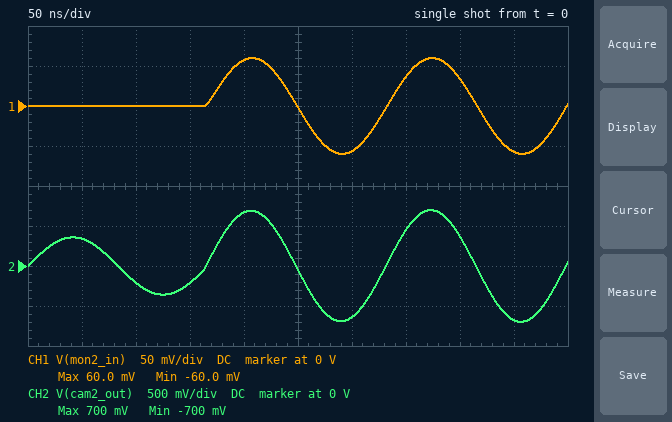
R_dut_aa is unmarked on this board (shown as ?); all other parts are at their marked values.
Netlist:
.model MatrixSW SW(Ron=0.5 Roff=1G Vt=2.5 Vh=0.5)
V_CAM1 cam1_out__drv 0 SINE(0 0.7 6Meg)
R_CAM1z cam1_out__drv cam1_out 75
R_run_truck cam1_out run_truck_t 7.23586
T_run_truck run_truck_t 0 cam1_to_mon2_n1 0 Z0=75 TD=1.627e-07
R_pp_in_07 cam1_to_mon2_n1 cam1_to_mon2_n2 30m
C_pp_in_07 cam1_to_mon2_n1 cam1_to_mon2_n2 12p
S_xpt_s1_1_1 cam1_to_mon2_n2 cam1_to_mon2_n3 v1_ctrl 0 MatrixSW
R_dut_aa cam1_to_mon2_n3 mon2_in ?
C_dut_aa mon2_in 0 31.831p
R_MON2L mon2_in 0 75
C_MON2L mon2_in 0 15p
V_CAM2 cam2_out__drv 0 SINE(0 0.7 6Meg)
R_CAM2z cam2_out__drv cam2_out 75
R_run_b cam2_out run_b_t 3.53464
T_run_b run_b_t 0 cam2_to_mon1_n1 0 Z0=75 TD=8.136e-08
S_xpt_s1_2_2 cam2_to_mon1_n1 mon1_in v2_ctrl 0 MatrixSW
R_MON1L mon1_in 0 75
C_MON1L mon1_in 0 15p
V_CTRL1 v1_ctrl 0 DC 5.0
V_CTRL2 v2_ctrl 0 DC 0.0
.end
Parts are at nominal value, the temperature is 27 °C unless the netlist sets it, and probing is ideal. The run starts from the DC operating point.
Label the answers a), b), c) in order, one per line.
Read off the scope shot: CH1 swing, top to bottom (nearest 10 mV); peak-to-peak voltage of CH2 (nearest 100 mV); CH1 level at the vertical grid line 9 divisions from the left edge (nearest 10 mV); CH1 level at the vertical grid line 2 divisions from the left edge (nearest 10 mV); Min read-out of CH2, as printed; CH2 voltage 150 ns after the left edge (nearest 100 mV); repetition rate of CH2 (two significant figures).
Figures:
a) 120 mV
b) 1.4 V
c) -60 mV
d) 0 V
e) -700 mV
f) -200 mV
g) 6.0 MHz
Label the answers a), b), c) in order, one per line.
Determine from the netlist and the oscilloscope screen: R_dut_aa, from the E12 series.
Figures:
a) 680 Ω
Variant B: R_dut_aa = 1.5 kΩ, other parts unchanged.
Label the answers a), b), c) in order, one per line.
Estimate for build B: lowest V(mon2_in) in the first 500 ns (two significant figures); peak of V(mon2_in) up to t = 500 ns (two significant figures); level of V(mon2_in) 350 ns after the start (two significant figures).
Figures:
a) -30 mV
b) 30 mV
c) 18 mV
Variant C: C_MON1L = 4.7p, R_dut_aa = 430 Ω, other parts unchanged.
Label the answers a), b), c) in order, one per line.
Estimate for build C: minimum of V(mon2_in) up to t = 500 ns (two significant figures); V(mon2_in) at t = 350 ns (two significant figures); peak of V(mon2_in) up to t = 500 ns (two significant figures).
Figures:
a) -86 mV
b) 53 mV
c) 86 mV
